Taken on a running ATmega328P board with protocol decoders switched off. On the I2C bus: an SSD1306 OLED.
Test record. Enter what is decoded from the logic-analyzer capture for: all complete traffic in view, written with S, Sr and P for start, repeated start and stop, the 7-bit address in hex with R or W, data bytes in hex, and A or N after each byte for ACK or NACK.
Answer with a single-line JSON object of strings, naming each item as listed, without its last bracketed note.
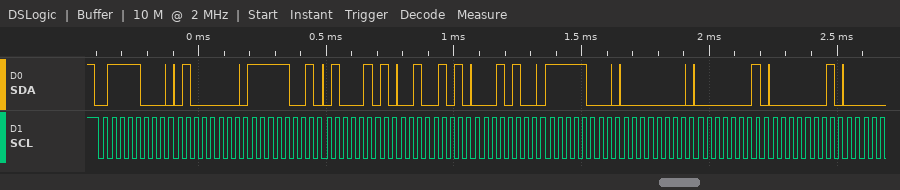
{"all complete traffic in view, written with S, Sr and P for start, repeated start and stop, the 7-bit address in hex with R or W, data bytes in hex, and A or N after each byte for ACK or NACK": "S 3CW A 40 A F9 A 45 A 25 A 14 A F8 A 00 A 01 A 01 A"}
